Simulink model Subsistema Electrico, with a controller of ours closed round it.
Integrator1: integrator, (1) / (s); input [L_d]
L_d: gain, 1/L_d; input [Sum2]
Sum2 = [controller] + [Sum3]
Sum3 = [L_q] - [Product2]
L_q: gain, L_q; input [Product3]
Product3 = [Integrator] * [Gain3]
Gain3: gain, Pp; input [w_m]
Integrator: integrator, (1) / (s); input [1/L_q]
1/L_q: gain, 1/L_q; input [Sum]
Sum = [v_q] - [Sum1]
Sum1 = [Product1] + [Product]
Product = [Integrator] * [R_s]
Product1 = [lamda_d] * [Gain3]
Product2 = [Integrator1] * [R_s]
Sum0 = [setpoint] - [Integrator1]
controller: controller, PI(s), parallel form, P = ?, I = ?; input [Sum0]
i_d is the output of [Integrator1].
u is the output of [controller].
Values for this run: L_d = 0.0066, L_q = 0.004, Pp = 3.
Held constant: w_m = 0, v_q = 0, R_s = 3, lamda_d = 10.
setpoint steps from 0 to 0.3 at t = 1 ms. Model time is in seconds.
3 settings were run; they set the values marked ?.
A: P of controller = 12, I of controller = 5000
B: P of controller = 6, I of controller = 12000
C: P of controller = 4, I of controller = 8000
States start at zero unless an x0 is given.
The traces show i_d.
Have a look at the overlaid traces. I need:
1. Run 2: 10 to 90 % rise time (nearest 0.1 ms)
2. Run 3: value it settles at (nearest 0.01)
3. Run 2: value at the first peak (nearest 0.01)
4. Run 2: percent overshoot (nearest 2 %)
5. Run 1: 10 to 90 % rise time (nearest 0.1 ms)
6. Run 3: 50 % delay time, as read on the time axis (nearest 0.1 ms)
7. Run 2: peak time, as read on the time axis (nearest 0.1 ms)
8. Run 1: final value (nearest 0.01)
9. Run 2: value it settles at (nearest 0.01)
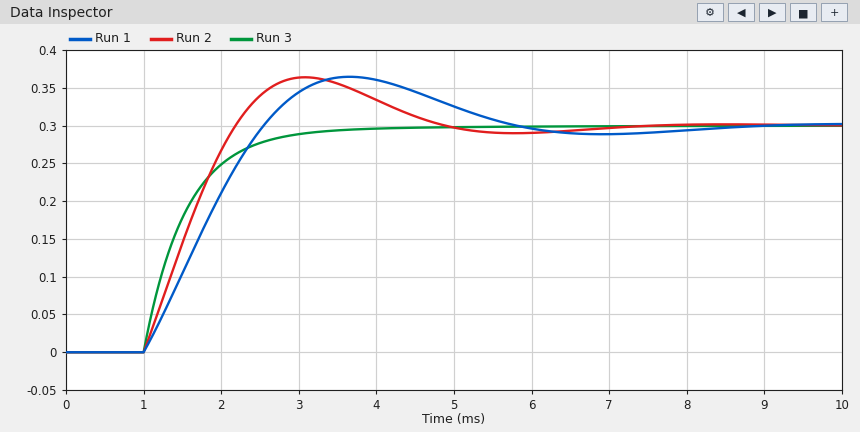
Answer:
0.9 ms
0.30
0.36
22 %
1.2 ms
1.4 ms
3.1 ms
0.30
0.30
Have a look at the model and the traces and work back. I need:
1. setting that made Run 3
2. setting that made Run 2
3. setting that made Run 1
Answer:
A
B
C
